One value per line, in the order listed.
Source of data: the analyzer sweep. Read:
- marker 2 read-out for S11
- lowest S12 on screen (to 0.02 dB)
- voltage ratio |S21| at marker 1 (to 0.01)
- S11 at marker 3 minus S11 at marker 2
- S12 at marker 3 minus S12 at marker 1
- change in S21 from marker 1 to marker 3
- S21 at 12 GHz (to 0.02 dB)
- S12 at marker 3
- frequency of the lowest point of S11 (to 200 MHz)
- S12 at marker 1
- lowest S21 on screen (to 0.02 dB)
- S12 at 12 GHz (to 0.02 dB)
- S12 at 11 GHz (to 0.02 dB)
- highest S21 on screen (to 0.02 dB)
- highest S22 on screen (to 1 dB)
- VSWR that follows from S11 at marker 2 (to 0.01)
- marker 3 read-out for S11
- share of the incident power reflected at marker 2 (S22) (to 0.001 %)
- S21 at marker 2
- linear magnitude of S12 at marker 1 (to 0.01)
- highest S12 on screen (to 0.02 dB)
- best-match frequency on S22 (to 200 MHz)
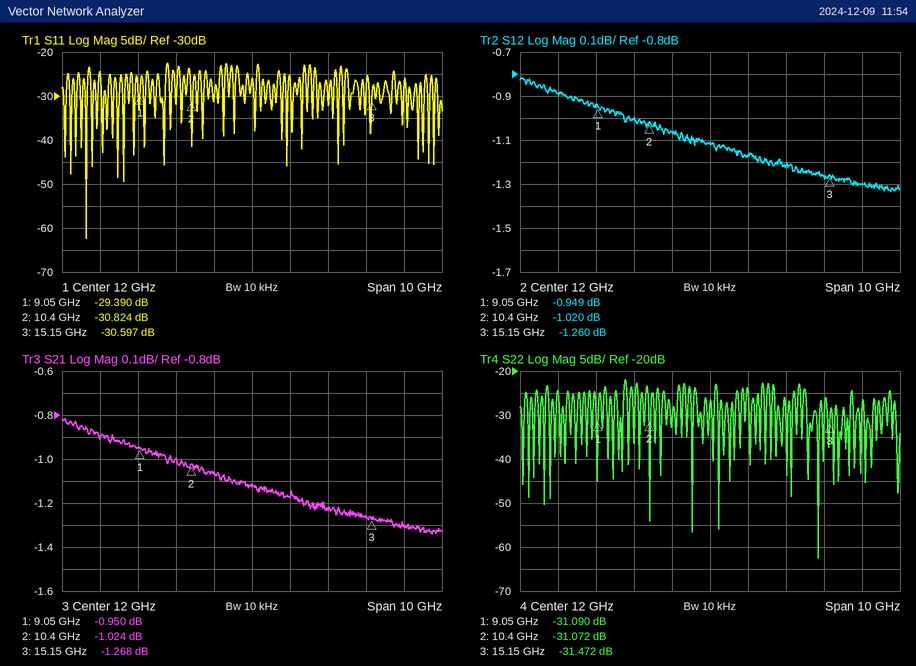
-30.824 dB
-1.34 dB
0.90
0.227 dB
-0.311 dB
-0.318 dB
-1.12 dB
-1.260 dB
7.6 GHz
-0.949 dB
-1.34 dB
-1.12 dB
-1.06 dB
-0.82 dB
-22 dB
1.06
-30.597 dB
0.078 %
-1.024 dB
0.90
-0.82 dB
14.8 GHz
